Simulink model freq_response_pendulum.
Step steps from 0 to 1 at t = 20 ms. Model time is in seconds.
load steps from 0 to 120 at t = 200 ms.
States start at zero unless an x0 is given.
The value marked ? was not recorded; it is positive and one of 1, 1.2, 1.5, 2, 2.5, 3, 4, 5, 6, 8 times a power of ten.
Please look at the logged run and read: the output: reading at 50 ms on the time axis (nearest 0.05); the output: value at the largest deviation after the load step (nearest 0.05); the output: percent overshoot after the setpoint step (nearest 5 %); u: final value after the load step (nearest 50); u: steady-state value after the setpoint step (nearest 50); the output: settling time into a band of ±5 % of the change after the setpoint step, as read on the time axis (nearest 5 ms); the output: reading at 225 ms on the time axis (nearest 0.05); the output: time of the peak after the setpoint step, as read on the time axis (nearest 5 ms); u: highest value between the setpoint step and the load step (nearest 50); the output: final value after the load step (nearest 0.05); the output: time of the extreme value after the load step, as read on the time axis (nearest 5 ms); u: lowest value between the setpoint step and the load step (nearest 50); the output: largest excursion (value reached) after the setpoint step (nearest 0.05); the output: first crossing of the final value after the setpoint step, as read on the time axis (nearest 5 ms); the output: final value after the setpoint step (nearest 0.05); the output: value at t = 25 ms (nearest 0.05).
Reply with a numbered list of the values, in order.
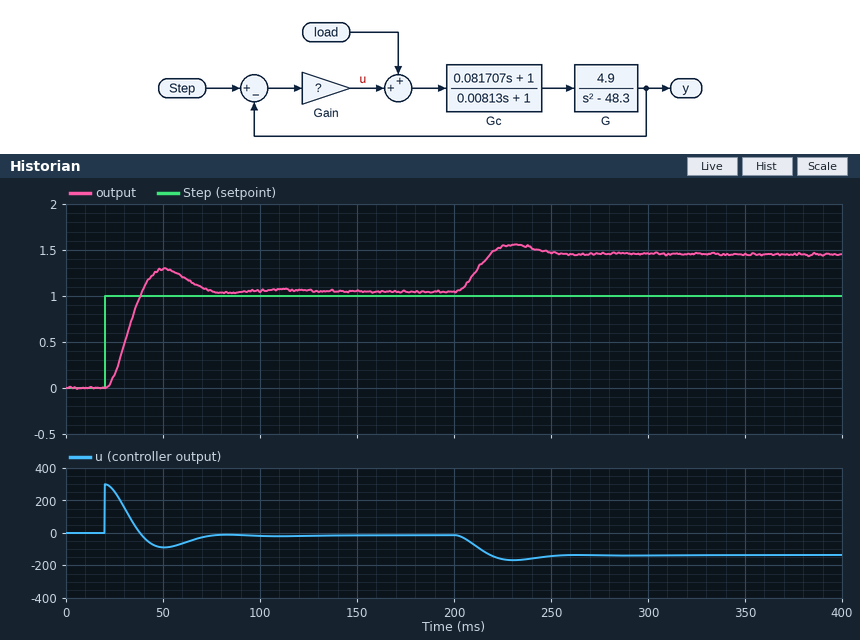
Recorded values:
1. 1.30
2. 1.55
3. 25 %
4. -150
5. 0
6. 70 ms
7. 1.55
8. 50 ms
9. 300
10. 1.45
11. 230 ms
12. -100
13. 1.30
14. 40 ms
15. 1.05
16. 0.15
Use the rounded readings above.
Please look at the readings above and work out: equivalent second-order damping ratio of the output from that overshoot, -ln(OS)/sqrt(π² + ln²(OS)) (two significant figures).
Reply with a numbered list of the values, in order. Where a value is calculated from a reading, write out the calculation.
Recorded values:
1. ln(0.25) = -1.386; 1.386 / sqrt(9.870 + 1.922) = 0.40
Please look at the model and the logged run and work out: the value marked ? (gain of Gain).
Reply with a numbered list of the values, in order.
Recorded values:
1. 300
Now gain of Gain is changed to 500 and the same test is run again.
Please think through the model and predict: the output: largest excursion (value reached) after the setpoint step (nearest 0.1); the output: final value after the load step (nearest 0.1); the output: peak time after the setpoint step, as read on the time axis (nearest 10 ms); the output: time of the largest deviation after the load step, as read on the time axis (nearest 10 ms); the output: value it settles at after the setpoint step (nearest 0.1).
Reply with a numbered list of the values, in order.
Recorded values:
1. 1.4
2. 1.3
3. 40 ms
4. 220 ms
5. 1.0
